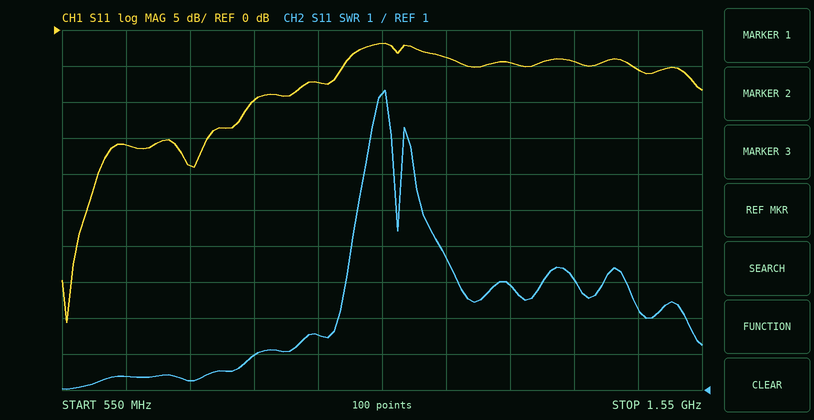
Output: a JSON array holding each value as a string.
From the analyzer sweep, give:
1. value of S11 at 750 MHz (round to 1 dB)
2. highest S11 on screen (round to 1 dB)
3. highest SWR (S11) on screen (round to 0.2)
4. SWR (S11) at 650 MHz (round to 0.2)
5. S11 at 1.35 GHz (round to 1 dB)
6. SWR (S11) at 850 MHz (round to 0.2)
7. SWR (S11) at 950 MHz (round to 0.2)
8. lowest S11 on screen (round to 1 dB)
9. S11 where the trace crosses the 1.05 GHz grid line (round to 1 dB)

["-19 dB", "-2 dB", "9.4", "1.4", "-4 dB", "2.0", "2.6", "-41 dB", "-2 dB"]
